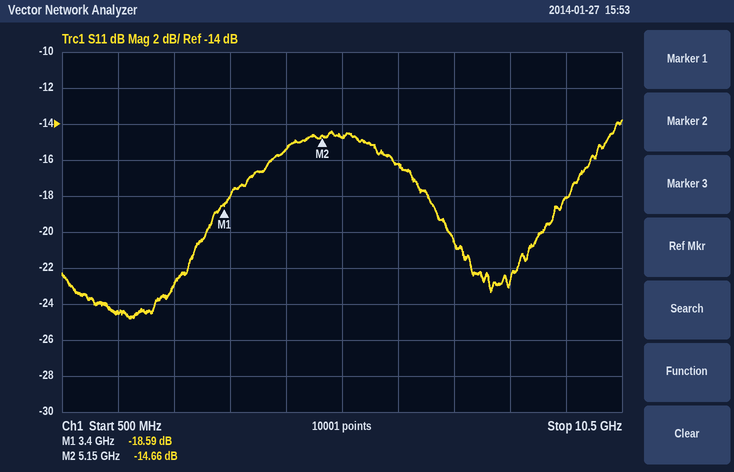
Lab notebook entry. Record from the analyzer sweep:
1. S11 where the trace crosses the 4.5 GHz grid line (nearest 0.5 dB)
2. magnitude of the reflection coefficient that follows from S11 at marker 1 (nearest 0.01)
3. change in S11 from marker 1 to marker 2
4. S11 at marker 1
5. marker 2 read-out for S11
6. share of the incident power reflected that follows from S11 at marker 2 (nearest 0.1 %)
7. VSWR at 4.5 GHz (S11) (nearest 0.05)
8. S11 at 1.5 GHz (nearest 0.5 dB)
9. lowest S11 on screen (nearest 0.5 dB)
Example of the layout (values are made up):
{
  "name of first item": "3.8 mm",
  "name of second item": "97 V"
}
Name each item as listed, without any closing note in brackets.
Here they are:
{
  "S11 where the trace crosses the 4.5 GHz grid line": "-15.5 dB",
  "magnitude of the reflection coefficient that follows from S11 at marker 1": "0.12",
  "change in S11 from marker 1 to marker 2": "3.93 dB",
  "S11 at marker 1": "-18.59 dB",
  "marker 2 read-out for S11": "-14.66 dB",
  "share of the incident power reflected that follows from S11 at marker 2": "3.4 %",
  "VSWR at 4.5 GHz (S11)": "1.40",
  "S11 at 1.5 GHz": "-24.5 dB",
  "lowest S11 on screen": "-25.0 dB"
}
